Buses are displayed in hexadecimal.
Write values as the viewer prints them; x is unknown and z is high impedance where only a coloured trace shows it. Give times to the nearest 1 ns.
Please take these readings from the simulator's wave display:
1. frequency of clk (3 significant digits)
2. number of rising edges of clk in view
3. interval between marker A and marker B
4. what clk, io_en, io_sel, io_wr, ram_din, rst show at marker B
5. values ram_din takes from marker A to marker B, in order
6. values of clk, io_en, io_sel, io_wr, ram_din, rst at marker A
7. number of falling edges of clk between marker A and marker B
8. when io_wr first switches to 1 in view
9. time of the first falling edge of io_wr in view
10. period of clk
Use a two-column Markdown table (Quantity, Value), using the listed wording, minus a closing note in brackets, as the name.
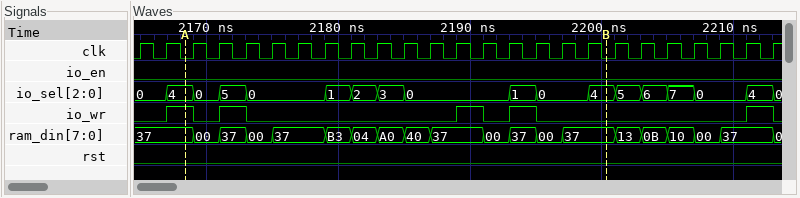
| Quantity | Value |
|---|---|
| frequency of clk | 500 MHz |
| number of rising edges of clk in view | 25 |
| interval between marker A and marker B | 32 ns |
| what clk, io_en, io_sel, io_wr, ram_din, rst show at marker B | clk=0, io_en=0, io_sel=4, io_wr=0, ram_din=37, rst=0 |
| values ram_din takes from marker A to marker B, in order | 37, 00, 37, 00, 37, B3, 04, A0, 40, 37, 00, 37, 00, 37 |
| values of clk, io_en, io_sel, io_wr, ram_din, rst at marker A | clk=0, io_en=0, io_sel=4, io_wr=1, ram_din=37, rst=0 |
| number of falling edges of clk between marker A and marker B | 16 |
| when io_wr first switches to 1 in view | 2167 ns |
| time of the first falling edge of io_wr in view | 2169 ns |
| period of clk | 2 ns |
